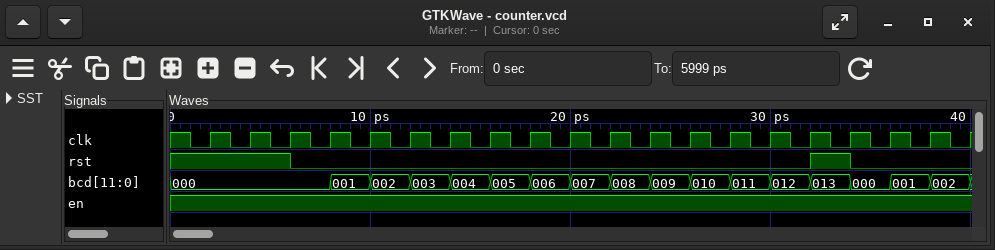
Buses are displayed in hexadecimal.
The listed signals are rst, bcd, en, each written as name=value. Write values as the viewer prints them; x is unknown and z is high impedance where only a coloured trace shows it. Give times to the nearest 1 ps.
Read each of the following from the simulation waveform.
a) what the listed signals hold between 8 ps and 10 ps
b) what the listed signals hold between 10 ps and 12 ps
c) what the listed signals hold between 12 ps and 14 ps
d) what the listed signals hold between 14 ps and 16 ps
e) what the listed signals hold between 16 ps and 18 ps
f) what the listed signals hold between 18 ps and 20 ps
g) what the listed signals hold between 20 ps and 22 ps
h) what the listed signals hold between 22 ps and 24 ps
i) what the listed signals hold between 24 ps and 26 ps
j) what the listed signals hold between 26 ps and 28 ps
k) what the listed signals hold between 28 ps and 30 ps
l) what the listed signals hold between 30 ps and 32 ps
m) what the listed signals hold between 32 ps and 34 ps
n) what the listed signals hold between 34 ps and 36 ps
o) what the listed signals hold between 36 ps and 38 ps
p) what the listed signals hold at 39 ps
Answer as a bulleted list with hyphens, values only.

- rst=0, bcd=001, en=1
- rst=0, bcd=002, en=1
- rst=0, bcd=003, en=1
- rst=0, bcd=004, en=1
- rst=0, bcd=005, en=1
- rst=0, bcd=006, en=1
- rst=0, bcd=007, en=1
- rst=0, bcd=008, en=1
- rst=0, bcd=009, en=1
- rst=0, bcd=010, en=1
- rst=0, bcd=011, en=1
- rst=0, bcd=012, en=1
- rst=1, bcd=013, en=1
- rst=0, bcd=000, en=1
- rst=0, bcd=001, en=1
- rst=0, bcd=002, en=1
